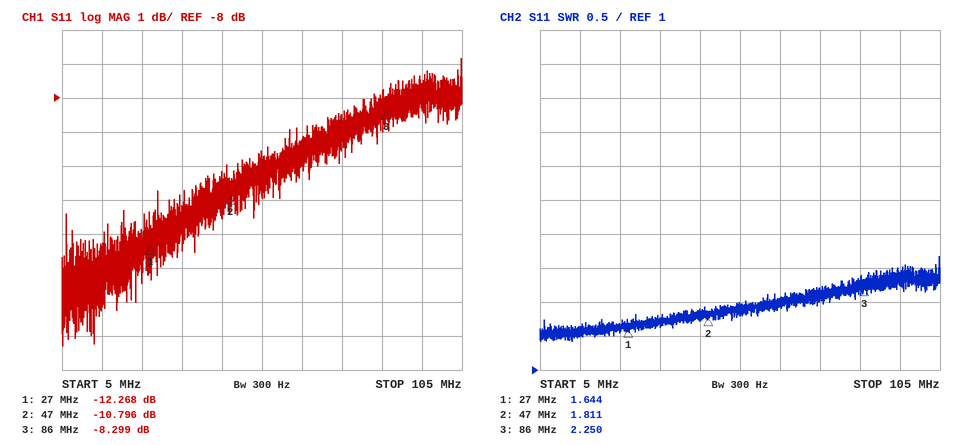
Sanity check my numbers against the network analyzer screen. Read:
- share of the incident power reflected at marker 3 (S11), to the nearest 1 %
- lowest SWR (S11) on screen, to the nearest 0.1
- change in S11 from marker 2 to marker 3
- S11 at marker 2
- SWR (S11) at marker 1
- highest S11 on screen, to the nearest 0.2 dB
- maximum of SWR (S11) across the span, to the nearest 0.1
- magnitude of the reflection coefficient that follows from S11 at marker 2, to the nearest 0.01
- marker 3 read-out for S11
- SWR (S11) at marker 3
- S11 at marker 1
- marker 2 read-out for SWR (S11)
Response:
15 %
1.4
2.497 dB
-10.796 dB
1.644
-6.8 dB
2.7
0.29
-8.299 dB
2.250
-12.268 dB
1.811
